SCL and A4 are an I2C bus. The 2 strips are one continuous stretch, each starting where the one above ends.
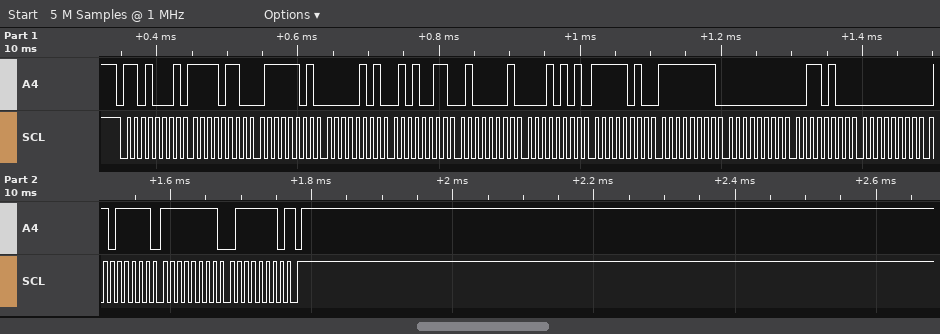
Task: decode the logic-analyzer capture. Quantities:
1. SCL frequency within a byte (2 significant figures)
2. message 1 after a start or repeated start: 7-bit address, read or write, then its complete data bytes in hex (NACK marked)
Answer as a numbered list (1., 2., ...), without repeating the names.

1. 100 kHz
2. 0x68 read: F6 7D 05 53 41 15 FA FF 00 34 00 5F FF 7E NACK
